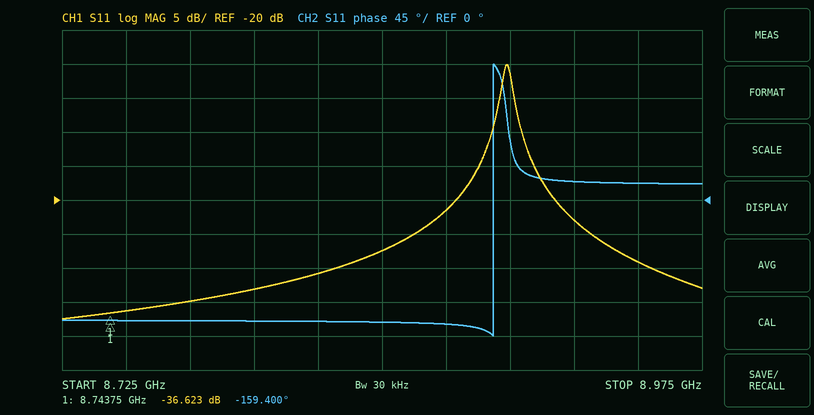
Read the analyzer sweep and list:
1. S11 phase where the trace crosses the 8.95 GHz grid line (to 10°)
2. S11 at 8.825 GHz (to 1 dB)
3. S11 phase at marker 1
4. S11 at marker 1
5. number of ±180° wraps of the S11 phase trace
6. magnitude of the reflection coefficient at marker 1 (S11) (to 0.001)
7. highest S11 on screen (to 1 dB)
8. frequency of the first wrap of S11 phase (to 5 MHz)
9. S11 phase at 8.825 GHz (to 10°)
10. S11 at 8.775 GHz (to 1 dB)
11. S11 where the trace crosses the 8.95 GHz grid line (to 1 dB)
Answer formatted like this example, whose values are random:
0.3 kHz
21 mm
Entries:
20°
-31 dB
-159.400°
-36.623 dB
1
0.015
0 dB
8.895 GHz
-160°
-35 dB
-29 dB
